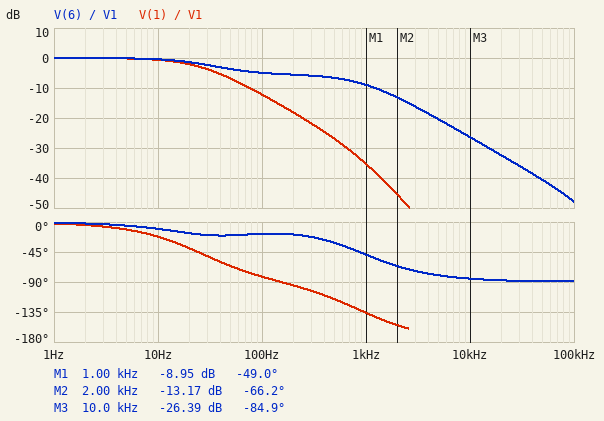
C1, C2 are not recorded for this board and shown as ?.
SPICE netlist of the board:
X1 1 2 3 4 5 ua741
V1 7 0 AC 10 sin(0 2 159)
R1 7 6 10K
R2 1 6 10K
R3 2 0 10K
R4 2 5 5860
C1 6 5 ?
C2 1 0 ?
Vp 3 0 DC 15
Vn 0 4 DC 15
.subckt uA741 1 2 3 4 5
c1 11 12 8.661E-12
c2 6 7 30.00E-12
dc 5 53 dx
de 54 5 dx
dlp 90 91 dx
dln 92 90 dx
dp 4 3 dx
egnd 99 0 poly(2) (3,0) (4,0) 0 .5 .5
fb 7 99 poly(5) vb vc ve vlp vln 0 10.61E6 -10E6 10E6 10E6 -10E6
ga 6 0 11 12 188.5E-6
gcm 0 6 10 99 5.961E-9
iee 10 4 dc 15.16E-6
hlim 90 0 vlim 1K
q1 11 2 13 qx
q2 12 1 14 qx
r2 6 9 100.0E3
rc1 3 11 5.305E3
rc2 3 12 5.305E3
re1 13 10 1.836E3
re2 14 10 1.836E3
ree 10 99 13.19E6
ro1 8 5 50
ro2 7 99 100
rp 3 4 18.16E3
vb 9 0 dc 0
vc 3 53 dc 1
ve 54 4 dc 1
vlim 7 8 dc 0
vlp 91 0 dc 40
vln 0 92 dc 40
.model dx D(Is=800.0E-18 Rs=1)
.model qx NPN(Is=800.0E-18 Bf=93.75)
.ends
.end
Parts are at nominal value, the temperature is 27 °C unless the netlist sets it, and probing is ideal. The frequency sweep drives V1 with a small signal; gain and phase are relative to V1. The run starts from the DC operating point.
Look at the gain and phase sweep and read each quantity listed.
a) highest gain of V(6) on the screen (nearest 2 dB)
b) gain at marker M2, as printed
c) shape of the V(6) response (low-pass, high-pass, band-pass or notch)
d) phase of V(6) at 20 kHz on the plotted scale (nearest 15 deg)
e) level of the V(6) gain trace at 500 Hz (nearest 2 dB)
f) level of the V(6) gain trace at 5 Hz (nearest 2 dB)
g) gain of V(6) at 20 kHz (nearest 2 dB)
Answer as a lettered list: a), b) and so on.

a) 0 dB
b) -13.17 dB
c) low-pass
d) -90 deg
e) -6 dB
f) 0 dB
g) -32 dB
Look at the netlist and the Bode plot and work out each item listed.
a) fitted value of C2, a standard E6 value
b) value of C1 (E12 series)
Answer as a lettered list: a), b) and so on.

a) 330 nF
b) 33 nF
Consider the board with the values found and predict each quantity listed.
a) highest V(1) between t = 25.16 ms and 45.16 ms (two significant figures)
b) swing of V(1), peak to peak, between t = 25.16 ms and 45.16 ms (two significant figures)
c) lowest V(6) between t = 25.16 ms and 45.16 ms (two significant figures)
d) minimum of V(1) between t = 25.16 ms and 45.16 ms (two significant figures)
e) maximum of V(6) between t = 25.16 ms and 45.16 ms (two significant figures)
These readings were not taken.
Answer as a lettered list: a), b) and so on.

a) 310 mV
b) 630 mV
c) -1.1 V
d) -310 mV
e) 1.1 V
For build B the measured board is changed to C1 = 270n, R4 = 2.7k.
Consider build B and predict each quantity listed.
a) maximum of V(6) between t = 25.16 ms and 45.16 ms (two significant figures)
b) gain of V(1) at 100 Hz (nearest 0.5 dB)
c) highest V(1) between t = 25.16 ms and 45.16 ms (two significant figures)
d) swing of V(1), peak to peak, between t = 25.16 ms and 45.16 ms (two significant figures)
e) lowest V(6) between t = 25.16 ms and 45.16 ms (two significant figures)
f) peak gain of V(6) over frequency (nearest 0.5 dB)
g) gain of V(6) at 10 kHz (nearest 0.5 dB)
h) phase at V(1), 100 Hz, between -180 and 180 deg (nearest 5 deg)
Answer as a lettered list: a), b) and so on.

a) 700 mV
b) -13.0 dB
c) 200 mV
d) 410 mV
e) -700 mV
f) 0 dB
g) -44.5 dB
h) -125 deg
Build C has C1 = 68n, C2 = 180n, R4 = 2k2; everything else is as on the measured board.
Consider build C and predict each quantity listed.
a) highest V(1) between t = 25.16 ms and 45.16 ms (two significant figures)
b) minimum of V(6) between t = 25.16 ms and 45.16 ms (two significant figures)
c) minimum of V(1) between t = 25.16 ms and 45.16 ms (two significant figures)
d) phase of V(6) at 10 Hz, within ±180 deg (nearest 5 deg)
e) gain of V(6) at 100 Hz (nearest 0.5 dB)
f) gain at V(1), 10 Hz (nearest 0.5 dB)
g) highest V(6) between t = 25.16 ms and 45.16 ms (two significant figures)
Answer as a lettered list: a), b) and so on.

a) 580 mV
b) -1.2 V
c) -580 mV
d) -5 deg
e) -3.5 dB
f) 0 dB
g) 1.2 V
